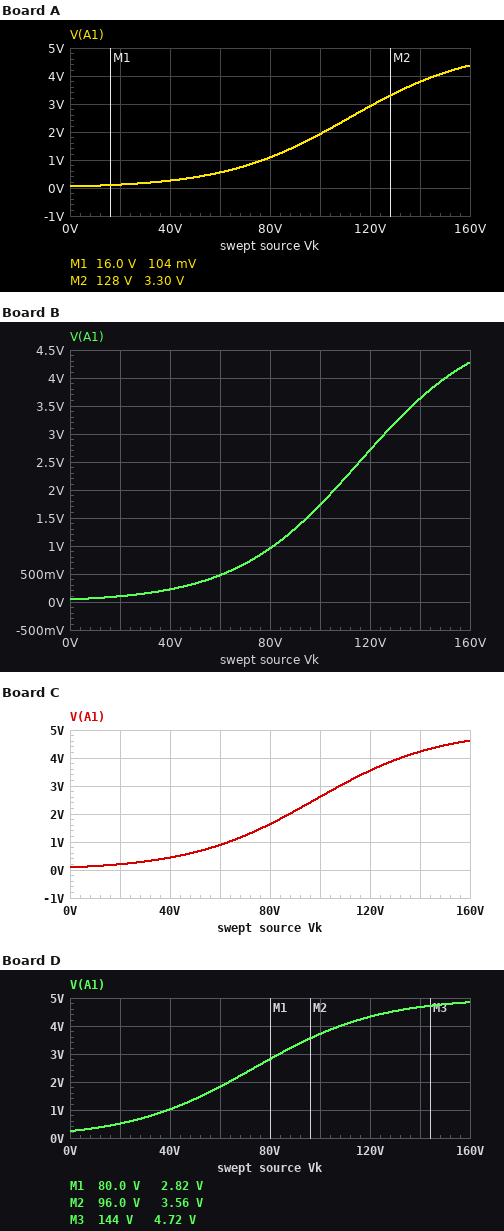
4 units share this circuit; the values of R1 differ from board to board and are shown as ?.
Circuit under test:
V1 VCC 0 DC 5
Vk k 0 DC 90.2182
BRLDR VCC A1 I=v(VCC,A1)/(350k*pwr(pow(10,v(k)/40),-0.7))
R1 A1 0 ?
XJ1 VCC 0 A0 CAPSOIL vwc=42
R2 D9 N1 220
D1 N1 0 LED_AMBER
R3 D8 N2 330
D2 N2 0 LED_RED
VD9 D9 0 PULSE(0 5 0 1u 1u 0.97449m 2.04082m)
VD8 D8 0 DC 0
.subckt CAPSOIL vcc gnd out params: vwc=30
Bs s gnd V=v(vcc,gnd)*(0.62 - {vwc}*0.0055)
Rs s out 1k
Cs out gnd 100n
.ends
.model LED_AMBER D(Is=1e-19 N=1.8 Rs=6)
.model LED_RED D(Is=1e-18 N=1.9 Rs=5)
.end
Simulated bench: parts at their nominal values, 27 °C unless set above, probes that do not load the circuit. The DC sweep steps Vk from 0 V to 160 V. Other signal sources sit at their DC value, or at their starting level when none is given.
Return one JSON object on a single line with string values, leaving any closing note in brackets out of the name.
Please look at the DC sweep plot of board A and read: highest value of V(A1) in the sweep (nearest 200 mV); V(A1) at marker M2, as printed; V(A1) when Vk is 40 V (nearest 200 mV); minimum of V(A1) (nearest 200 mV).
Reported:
{"highest value of V(A1) in the sweep": "4.4 V", "V(A1) at marker M2, as printed": "3.30 V", "V(A1) when Vk is 40 V": "200 mV", "minimum of V(A1)": "0 V"}
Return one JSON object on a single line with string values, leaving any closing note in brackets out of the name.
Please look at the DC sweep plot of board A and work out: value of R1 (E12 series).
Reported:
{"value of R1": "3.9 kΩ"}
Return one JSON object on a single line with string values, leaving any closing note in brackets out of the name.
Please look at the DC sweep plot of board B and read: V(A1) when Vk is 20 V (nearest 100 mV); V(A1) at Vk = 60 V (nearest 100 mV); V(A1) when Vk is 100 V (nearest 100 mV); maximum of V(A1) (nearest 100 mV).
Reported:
{"V(A1) when Vk is 20 V": "100 mV", "V(A1) at Vk = 60 V": "500 mV", "V(A1) when Vk is 100 V": "1.7 V", "maximum of V(A1)": "4.3 V"}
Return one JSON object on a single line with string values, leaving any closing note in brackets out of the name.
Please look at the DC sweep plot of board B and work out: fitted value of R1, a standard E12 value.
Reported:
{"fitted value of R1, a standard E12 value": "3.3 kΩ"}
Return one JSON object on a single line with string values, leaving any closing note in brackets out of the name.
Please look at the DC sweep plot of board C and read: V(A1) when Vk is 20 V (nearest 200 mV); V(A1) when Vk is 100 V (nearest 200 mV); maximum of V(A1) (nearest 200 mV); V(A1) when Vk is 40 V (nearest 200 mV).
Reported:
{"V(A1) when Vk is 20 V": "200 mV", "V(A1) when Vk is 100 V": "2.6 V", "maximum of V(A1)": "4.6 V", "V(A1) when Vk is 40 V": "400 mV"}
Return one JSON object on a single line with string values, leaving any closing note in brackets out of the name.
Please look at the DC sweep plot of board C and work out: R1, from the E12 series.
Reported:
{"R1, from the E12 series": "6.8 kΩ"}
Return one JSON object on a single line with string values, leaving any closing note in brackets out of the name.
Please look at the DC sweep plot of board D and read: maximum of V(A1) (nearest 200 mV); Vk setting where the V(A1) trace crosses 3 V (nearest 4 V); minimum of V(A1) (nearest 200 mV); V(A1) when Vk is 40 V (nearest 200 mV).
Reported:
{"maximum of V(A1)": "4.8 V", "Vk setting where the V(A1) trace crosses 3 V": "84 V", "minimum of V(A1)": "200 mV", "V(A1) when Vk is 40 V": "1.0 V"}
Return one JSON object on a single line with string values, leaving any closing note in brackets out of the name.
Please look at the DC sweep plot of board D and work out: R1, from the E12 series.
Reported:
{"R1, from the E12 series": "18 kΩ"}
